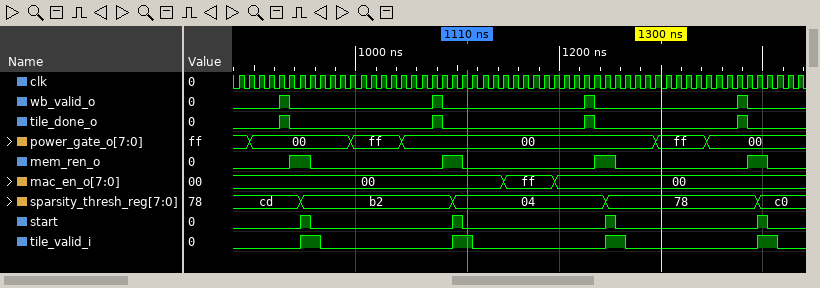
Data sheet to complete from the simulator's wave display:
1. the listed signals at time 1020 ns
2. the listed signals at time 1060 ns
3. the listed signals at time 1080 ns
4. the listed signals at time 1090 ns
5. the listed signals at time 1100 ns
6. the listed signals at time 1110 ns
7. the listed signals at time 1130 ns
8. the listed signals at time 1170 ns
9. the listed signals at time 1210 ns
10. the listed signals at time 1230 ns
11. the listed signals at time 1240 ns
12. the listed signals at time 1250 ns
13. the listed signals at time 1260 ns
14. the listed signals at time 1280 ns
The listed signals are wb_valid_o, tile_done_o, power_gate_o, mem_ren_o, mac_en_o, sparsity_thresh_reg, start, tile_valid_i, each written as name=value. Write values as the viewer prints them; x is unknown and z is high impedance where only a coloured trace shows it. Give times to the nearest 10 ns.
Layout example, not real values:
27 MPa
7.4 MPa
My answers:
wb_valid_o=0, tile_done_o=0, power_gate_o=ff, mem_ren_o=0, mac_en_o=00, sparsity_thresh_reg=b2, start=0, tile_valid_i=0
wb_valid_o=0, tile_done_o=0, power_gate_o=00, mem_ren_o=0, mac_en_o=00, sparsity_thresh_reg=b2, start=0, tile_valid_i=0
wb_valid_o=1, tile_done_o=1, power_gate_o=00, mem_ren_o=0, mac_en_o=00, sparsity_thresh_reg=b2, start=0, tile_valid_i=0
wb_valid_o=0, tile_done_o=0, power_gate_o=00, mem_ren_o=1, mac_en_o=00, sparsity_thresh_reg=b2, start=0, tile_valid_i=0
wb_valid_o=0, tile_done_o=0, power_gate_o=00, mem_ren_o=1, mac_en_o=00, sparsity_thresh_reg=04, start=1, tile_valid_i=1
wb_valid_o=0, tile_done_o=0, power_gate_o=00, mem_ren_o=0, mac_en_o=00, sparsity_thresh_reg=04, start=0, tile_valid_i=1
wb_valid_o=0, tile_done_o=0, power_gate_o=00, mem_ren_o=0, mac_en_o=00, sparsity_thresh_reg=04, start=0, tile_valid_i=0
wb_valid_o=0, tile_done_o=0, power_gate_o=00, mem_ren_o=0, mac_en_o=ff, sparsity_thresh_reg=04, start=0, tile_valid_i=0
wb_valid_o=0, tile_done_o=0, power_gate_o=00, mem_ren_o=0, mac_en_o=00, sparsity_thresh_reg=04, start=0, tile_valid_i=0
wb_valid_o=1, tile_done_o=1, power_gate_o=00, mem_ren_o=0, mac_en_o=00, sparsity_thresh_reg=04, start=0, tile_valid_i=0
wb_valid_o=0, tile_done_o=0, power_gate_o=00, mem_ren_o=1, mac_en_o=00, sparsity_thresh_reg=04, start=0, tile_valid_i=0
wb_valid_o=0, tile_done_o=0, power_gate_o=00, mem_ren_o=1, mac_en_o=00, sparsity_thresh_reg=78, start=1, tile_valid_i=1
wb_valid_o=0, tile_done_o=0, power_gate_o=00, mem_ren_o=0, mac_en_o=00, sparsity_thresh_reg=78, start=0, tile_valid_i=1
wb_valid_o=0, tile_done_o=0, power_gate_o=00, mem_ren_o=0, mac_en_o=00, sparsity_thresh_reg=78, start=0, tile_valid_i=0
